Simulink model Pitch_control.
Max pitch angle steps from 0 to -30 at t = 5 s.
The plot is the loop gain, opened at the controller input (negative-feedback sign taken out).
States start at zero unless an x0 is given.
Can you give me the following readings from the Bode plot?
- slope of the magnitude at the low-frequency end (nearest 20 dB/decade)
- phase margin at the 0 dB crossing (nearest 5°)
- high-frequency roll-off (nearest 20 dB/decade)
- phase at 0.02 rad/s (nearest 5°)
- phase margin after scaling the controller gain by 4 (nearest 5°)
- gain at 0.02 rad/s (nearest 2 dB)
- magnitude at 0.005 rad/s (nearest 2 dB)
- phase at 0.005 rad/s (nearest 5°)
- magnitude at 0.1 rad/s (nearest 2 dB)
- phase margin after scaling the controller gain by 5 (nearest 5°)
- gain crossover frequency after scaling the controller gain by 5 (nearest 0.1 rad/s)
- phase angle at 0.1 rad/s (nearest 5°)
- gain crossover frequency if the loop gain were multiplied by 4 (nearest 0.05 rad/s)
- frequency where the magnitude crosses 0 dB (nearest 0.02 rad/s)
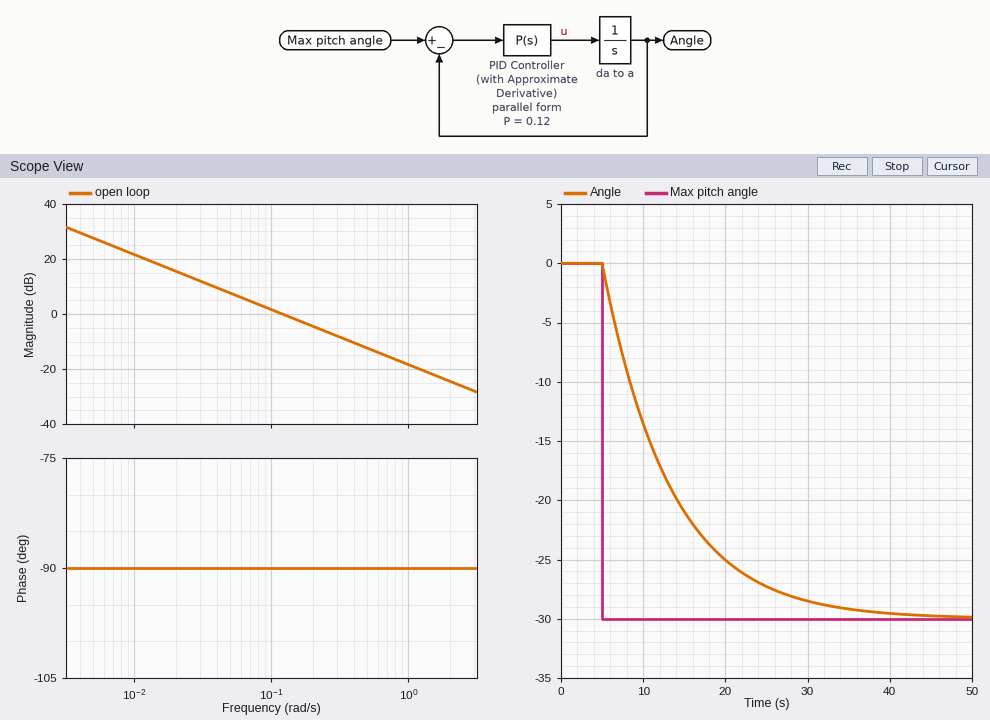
-20 dB/decade
90°
-20 dB/decade
-90°
90°
16 dB
28 dB
-90°
2 dB
90°
0.6 rad/s
-90°
0.50 rad/s
0.12 rad/s
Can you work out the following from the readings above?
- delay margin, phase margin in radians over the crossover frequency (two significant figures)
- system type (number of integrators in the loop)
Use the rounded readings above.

13 s
1
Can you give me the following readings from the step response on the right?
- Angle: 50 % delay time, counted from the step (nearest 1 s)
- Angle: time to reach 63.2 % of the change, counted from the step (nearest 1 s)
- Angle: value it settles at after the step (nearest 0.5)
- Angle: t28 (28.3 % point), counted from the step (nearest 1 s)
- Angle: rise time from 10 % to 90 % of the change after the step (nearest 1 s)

6 s
8 s
-30.0
3 s
18 s
